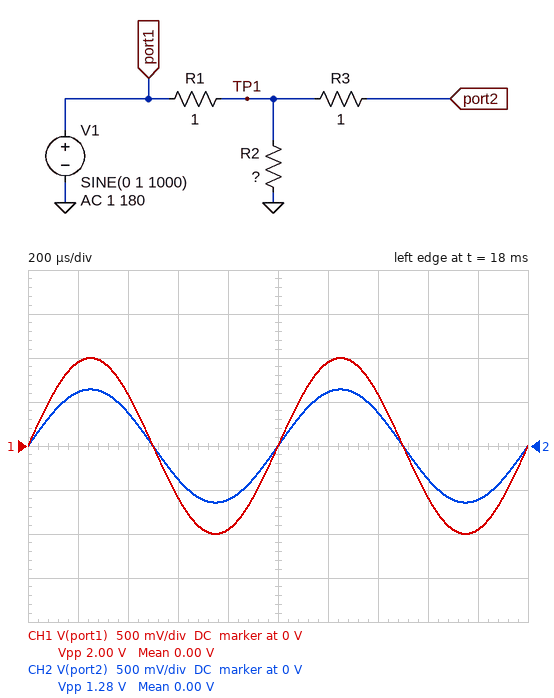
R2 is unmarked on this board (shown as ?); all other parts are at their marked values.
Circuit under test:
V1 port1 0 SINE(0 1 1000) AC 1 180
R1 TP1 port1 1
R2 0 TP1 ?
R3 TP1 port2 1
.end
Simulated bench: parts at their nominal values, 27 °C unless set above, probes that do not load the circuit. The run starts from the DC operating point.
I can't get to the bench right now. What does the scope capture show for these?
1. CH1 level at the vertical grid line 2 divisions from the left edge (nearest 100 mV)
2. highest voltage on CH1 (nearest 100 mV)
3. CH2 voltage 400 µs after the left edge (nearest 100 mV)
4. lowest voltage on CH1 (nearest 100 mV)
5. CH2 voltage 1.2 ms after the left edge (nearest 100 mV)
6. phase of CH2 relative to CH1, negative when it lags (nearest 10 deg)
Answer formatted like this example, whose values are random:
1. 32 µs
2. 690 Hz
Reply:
1. 600 mV
2. 1.0 V
3. 400 mV
4. -1.0 V
5. 600 mV
6. 0 deg
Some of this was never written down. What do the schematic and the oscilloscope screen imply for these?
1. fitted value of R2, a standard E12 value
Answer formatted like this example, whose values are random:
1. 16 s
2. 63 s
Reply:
1. 1.8 Ω
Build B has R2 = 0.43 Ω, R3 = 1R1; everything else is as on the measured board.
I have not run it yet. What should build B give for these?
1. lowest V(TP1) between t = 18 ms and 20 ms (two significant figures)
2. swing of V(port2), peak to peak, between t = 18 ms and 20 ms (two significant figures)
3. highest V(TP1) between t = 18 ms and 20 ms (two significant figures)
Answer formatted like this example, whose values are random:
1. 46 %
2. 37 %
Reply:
1. -300 mV
2. 600 mV
3. 300 mV
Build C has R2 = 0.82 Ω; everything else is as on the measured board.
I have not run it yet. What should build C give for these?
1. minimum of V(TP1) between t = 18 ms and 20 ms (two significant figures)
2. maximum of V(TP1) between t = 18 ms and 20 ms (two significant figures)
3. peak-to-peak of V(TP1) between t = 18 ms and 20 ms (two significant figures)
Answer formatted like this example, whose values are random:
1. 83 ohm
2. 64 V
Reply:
1. -450 mV
2. 450 mV
3. 900 mV
